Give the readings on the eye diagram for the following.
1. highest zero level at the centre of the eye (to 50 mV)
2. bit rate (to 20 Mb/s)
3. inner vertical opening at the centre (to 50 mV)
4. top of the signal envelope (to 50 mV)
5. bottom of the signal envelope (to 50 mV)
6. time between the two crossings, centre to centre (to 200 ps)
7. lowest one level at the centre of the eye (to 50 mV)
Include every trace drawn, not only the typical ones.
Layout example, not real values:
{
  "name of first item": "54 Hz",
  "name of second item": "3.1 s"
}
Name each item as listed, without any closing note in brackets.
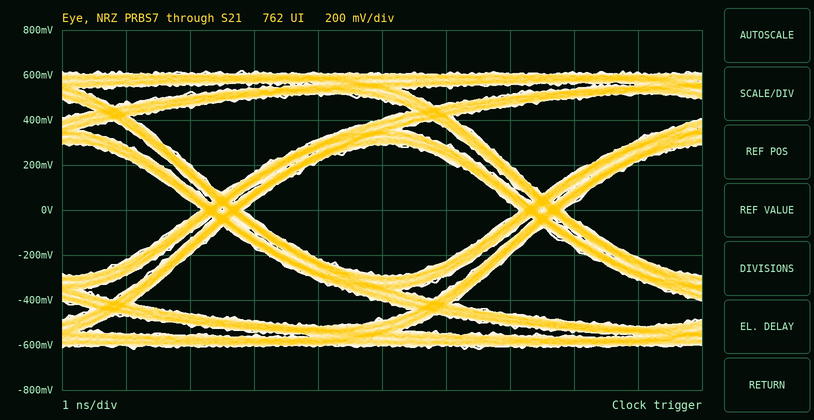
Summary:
{
  "highest zero level at the centre of the eye": "-300 mV",
  "bit rate": "200 Mb/s",
  "inner vertical opening at the centre": "600 mV",
  "top of the signal envelope": "600 mV",
  "bottom of the signal envelope": "-600 mV",
  "time between the two crossings, centre to centre": "5.0 ns",
  "lowest one level at the centre of the eye": "300 mV"
}
